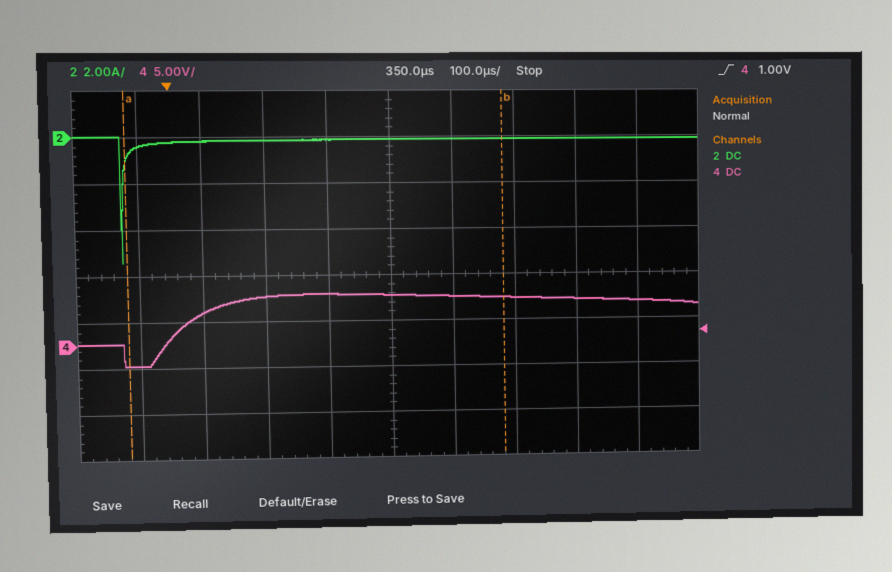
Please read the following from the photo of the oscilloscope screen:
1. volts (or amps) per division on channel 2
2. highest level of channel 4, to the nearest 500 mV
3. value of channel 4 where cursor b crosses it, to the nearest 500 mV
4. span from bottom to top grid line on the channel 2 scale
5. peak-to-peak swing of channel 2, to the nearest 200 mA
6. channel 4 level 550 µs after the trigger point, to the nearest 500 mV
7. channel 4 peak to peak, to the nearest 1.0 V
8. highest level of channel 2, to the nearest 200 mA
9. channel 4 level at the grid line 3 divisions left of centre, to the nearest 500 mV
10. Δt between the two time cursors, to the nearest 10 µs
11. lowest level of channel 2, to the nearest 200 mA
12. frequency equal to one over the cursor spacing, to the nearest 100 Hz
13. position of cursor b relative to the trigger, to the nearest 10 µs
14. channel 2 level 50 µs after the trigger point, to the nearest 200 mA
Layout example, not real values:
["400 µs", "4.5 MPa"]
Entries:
["2 A", "5.5 V", "5.0 V", "16 A", "5.4 A", "5.0 V", "8.0 V", "0.0 A", "3.5 V", "600 µs", "-5.4 A", "1.7 kHz", "+530 µs", "-200 mA"]
